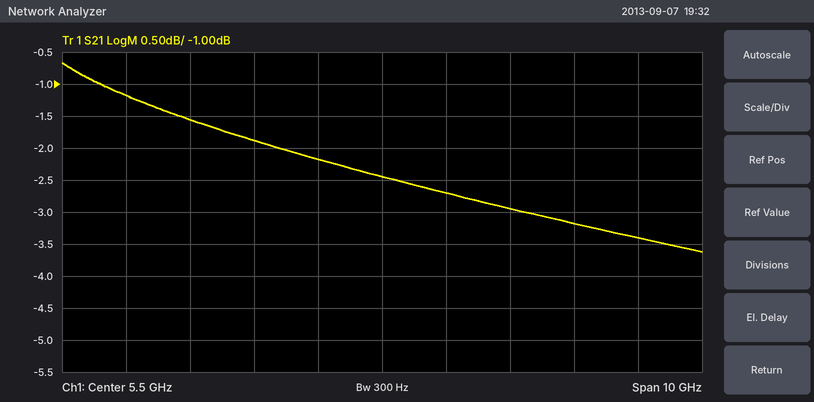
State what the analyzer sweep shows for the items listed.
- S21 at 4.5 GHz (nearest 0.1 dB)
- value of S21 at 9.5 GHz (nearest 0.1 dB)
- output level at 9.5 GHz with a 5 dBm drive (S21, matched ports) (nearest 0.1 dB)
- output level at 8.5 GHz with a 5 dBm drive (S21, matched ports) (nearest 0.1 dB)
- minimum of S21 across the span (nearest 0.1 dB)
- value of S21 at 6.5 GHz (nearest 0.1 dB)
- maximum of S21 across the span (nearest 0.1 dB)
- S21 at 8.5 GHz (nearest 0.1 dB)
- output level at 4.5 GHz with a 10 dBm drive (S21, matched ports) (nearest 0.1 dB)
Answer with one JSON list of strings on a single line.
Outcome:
["-2.2 dB", "-3.4 dB", "1.6 dBm", "1.8 dBm", "-3.6 dB", "-2.7 dB", "-0.7 dB", "-3.2 dB", "7.8 dBm"]
